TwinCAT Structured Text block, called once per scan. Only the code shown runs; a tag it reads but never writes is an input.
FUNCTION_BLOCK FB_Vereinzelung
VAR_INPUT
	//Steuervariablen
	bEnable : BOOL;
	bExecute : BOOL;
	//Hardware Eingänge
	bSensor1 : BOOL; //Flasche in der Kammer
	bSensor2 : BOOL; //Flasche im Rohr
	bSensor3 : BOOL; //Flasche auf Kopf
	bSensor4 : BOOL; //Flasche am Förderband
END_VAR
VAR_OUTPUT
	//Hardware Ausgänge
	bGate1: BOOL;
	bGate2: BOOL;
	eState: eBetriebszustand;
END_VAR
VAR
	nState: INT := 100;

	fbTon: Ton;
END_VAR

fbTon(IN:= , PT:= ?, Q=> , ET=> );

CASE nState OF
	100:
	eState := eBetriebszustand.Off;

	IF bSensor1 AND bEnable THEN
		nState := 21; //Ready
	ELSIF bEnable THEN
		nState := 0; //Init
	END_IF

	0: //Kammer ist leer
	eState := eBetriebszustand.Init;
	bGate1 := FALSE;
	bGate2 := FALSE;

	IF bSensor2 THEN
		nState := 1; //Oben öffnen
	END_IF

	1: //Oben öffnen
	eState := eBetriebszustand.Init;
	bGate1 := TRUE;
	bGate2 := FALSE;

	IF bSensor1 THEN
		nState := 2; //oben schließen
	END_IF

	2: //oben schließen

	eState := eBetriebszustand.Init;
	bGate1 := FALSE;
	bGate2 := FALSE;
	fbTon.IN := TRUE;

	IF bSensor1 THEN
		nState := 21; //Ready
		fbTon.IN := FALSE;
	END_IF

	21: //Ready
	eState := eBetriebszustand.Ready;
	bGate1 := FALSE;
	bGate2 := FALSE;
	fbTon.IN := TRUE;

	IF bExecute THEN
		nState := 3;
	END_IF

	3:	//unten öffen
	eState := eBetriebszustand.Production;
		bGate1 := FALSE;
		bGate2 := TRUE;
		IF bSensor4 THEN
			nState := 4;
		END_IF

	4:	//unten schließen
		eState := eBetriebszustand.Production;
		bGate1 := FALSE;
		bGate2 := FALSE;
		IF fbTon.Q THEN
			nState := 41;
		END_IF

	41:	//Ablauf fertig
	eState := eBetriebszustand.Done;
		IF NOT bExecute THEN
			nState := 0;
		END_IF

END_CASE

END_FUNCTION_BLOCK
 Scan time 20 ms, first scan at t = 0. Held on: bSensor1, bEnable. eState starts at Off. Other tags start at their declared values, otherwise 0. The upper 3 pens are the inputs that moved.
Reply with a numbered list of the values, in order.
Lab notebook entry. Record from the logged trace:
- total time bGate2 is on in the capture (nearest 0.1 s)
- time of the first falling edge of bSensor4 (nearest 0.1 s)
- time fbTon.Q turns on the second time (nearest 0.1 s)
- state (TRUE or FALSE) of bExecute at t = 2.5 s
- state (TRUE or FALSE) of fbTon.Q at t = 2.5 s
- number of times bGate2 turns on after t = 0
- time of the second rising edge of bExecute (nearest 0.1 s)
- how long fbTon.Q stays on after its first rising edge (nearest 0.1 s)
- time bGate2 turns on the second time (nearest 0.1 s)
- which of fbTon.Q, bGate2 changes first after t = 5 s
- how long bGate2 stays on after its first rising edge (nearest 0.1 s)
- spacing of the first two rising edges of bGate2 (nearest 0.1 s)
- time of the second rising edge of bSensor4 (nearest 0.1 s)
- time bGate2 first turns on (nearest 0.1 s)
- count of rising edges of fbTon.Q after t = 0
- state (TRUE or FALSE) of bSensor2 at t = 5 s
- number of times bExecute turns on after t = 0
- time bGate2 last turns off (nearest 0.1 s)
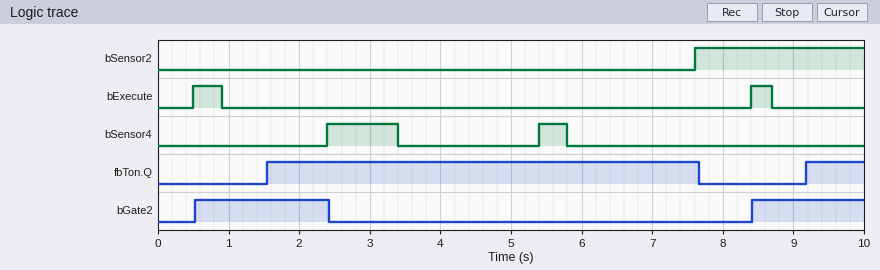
1. 3.5 s
2. 3.4 s
3. 9.2 s
4. FALSE
5. TRUE
6. 2
7. 8.4 s
8. 6.1 s
9. 8.4 s
10. fbTon.Q
11. 1.9 s
12. 7.9 s
13. 5.4 s
14. 0.5 s
15. 2
16. FALSE
17. 2
18. 2.4 s
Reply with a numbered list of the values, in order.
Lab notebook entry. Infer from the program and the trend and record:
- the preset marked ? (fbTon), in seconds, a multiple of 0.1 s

1. 1.5 s
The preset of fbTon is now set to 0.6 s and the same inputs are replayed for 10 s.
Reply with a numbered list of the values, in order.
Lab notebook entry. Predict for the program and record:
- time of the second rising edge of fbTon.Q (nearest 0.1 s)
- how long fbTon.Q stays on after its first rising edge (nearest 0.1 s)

1. 8.3 s
2. 7.0 s
